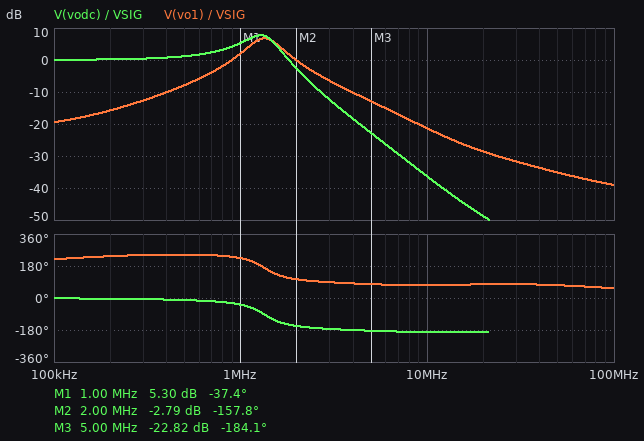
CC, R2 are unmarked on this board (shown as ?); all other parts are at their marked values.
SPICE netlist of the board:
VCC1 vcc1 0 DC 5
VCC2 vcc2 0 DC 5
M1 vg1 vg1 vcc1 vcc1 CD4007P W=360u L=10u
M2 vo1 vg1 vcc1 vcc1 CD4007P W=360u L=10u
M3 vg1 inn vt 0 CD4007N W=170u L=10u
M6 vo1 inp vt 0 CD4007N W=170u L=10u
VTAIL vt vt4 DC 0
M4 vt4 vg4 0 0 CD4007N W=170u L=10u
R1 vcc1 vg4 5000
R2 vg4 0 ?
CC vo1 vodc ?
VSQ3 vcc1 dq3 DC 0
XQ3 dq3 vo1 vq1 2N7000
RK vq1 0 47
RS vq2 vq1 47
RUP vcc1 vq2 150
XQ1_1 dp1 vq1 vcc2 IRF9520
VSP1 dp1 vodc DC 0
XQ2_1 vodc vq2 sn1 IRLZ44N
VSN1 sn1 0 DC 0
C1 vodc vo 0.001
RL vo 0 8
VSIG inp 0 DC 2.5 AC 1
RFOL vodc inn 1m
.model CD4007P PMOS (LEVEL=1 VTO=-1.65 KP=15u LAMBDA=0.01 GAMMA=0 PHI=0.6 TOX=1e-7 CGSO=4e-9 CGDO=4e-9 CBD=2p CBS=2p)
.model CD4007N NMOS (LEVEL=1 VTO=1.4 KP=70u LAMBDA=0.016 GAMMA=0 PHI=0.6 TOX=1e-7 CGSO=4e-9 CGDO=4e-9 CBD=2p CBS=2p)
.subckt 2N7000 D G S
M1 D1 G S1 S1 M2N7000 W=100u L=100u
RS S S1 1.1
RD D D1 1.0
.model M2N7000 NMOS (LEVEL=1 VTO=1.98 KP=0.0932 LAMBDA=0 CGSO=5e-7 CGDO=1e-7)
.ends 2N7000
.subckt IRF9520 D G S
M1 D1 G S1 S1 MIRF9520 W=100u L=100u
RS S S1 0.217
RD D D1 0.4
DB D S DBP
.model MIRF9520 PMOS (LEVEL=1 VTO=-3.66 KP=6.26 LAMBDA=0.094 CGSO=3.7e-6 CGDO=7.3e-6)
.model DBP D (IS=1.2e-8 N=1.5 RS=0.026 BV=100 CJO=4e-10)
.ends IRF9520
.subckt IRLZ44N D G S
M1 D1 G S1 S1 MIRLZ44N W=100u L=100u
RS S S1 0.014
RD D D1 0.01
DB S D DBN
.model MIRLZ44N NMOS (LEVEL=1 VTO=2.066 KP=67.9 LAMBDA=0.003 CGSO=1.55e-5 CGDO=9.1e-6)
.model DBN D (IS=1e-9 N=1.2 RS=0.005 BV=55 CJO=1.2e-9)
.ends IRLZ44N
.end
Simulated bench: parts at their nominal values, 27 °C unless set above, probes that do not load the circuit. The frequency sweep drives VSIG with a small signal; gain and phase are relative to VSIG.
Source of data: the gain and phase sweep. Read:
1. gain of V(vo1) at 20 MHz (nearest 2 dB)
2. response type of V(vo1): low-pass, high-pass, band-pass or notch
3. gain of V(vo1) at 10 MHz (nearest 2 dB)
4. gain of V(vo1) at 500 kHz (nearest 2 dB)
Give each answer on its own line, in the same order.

-28 dB
band-pass
-22 dB
-8 dB
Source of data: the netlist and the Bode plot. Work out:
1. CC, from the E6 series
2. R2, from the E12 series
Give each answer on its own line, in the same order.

33 pF
3.9 kΩ
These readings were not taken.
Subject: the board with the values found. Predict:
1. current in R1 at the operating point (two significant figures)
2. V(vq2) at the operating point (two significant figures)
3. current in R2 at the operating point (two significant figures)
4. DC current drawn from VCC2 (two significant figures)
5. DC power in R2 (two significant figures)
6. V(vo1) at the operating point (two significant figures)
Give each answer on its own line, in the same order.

560 µA
2.1 V
560 µA
60 mA
1.2 mW
3.6 V
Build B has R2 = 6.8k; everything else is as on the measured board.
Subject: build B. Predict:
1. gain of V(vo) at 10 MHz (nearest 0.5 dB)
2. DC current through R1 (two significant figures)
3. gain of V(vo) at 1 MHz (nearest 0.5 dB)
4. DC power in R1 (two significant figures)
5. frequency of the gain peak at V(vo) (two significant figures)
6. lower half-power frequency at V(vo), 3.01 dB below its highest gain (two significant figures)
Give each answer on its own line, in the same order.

-32.5 dB
420 µA
4.0 dB
900 µW
1.5 MHz
1.2 MHz
